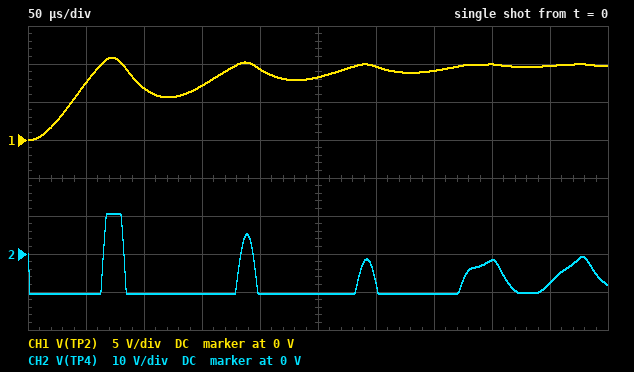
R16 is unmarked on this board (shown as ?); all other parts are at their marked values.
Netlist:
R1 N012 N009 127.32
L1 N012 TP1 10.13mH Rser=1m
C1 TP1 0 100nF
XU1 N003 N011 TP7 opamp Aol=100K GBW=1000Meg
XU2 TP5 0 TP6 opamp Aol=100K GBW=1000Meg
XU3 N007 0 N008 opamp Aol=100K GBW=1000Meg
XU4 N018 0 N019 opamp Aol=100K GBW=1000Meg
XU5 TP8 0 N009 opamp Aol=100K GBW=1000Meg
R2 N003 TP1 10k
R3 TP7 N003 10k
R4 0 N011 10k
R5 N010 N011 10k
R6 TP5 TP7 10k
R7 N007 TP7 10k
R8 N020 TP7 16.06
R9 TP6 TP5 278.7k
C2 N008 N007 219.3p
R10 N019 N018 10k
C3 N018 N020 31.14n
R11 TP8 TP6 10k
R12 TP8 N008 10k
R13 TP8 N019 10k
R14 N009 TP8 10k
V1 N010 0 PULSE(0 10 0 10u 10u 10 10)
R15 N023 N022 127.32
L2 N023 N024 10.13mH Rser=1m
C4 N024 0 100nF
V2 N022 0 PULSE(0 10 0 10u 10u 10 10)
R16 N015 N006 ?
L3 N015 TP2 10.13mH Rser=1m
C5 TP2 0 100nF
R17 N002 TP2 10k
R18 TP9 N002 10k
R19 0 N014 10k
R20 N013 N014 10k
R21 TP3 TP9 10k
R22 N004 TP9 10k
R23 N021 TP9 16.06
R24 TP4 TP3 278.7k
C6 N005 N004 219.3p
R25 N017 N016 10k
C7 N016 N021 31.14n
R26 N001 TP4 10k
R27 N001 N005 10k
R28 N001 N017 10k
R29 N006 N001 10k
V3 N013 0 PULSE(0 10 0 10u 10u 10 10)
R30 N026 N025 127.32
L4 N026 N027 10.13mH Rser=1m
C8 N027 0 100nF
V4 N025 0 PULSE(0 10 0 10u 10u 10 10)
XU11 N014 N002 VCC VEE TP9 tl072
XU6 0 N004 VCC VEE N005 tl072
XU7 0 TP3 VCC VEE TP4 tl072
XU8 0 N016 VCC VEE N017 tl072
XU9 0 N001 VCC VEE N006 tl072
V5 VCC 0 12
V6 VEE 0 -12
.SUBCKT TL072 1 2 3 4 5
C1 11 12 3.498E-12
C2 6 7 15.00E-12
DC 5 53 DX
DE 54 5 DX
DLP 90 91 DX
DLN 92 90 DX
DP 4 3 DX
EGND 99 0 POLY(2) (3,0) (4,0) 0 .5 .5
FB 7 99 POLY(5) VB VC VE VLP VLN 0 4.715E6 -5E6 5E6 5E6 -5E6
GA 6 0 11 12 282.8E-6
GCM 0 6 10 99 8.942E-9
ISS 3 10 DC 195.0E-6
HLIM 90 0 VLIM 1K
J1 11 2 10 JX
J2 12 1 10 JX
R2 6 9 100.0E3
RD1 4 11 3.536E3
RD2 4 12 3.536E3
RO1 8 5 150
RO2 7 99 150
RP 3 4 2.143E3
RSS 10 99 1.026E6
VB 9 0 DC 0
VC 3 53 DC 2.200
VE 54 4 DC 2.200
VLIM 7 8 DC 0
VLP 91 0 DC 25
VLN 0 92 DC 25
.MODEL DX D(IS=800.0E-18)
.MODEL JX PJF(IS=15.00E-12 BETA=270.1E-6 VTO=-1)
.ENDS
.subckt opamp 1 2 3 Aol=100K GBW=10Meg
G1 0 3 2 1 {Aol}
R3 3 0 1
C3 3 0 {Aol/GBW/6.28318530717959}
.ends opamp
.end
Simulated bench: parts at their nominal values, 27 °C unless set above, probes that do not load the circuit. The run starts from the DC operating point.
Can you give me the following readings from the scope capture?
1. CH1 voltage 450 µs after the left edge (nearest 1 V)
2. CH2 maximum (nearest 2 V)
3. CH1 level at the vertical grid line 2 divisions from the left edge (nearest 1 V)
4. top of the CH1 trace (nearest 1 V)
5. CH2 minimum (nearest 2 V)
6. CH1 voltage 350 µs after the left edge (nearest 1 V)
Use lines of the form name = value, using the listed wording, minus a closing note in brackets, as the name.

CH1 voltage 450 µs after the left edge = 10 V
CH2 maximum = 10 V
CH1 level at the vertical grid line 2 divisions from the left edge = 7 V
top of the CH1 trace = 11 V
CH2 minimum = -10 V
CH1 voltage 350 µs after the left edge = 9 V
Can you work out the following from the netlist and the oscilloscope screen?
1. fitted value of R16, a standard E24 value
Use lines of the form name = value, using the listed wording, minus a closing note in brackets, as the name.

fitted value of R16, a standard E24 value = 220 Ω
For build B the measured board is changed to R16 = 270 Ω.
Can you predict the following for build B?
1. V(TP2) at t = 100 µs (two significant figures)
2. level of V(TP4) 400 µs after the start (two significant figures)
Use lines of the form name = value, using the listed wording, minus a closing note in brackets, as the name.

V(TP2) at t = 100 µs = 7.7 V
level of V(TP4) 400 µs after the start = -6.5 V
